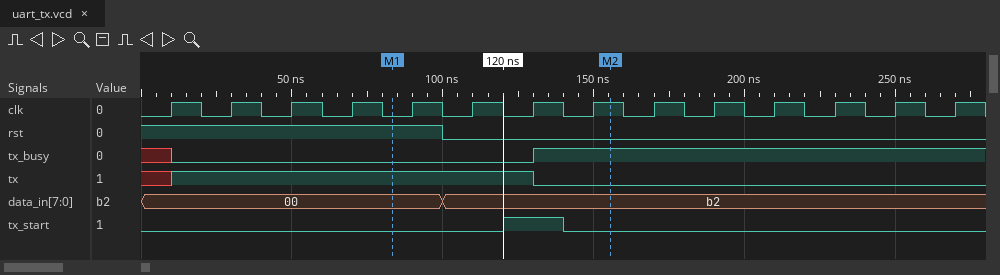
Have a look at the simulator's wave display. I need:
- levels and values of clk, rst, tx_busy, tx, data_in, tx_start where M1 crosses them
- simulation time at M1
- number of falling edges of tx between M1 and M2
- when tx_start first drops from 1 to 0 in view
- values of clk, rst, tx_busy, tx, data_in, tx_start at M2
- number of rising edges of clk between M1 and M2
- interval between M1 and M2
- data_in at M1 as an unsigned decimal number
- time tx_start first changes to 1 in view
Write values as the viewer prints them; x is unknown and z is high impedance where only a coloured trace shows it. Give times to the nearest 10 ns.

clk=0, rst=1, tx_busy=0, tx=1, data_in=00, tx_start=0
80 ns
1
140 ns
clk=1, rst=0, tx_busy=1, tx=0, data_in=b2, tx_start=0
4
70 ns
0
120 ns
